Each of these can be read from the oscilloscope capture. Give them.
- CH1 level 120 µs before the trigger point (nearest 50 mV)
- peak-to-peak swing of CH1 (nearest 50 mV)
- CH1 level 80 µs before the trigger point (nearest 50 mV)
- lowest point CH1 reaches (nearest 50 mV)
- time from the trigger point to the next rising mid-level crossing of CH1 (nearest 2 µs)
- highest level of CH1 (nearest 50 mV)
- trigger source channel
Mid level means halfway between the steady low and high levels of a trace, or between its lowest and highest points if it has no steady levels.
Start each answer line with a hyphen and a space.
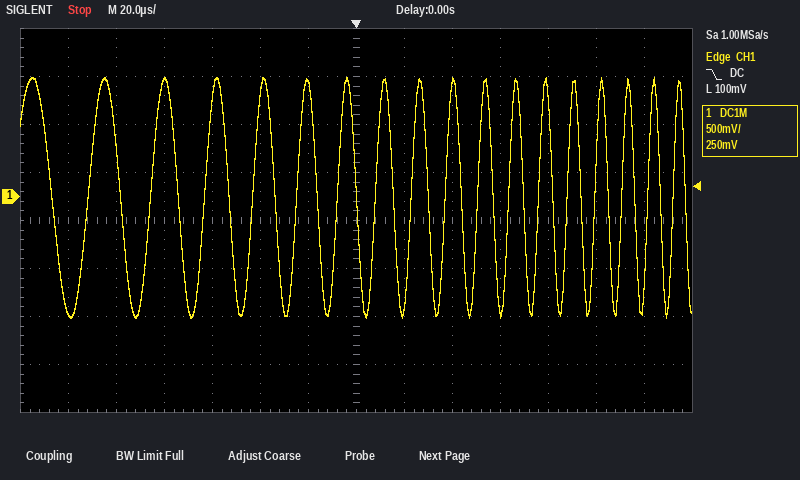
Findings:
- -1.20 V
- 2.50 V
- 1.20 V
- -1.25 V
- 8 µs
- 1.25 V
- CH1
